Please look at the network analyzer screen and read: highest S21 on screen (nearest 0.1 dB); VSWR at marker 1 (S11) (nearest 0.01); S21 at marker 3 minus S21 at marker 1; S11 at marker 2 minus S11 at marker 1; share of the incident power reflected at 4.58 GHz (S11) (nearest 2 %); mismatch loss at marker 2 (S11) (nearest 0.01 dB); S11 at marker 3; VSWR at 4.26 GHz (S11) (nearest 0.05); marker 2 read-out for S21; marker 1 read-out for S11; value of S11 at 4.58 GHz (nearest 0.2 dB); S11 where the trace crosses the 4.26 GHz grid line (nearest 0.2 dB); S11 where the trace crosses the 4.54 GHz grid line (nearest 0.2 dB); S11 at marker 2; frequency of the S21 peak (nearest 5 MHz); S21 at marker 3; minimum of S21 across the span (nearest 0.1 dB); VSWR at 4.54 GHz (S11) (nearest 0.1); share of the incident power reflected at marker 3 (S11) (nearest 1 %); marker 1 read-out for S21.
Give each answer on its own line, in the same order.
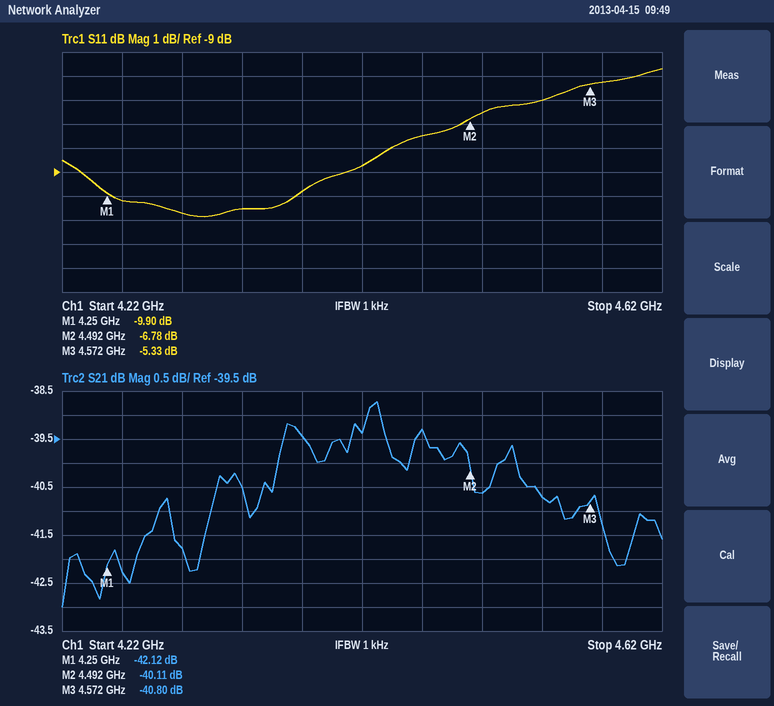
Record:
-38.7 dB
1.94
1.32 dB
3.12 dB
30 %
1.02 dB
-5.33 dB
1.90
-40.11 dB
-9.90 dB
-5.2 dB
-10.2 dB
-6.0 dB
-6.78 dB
4.430 GHz
-40.80 dB
-43.0 dB
3.0
29 %
-42.12 dB
